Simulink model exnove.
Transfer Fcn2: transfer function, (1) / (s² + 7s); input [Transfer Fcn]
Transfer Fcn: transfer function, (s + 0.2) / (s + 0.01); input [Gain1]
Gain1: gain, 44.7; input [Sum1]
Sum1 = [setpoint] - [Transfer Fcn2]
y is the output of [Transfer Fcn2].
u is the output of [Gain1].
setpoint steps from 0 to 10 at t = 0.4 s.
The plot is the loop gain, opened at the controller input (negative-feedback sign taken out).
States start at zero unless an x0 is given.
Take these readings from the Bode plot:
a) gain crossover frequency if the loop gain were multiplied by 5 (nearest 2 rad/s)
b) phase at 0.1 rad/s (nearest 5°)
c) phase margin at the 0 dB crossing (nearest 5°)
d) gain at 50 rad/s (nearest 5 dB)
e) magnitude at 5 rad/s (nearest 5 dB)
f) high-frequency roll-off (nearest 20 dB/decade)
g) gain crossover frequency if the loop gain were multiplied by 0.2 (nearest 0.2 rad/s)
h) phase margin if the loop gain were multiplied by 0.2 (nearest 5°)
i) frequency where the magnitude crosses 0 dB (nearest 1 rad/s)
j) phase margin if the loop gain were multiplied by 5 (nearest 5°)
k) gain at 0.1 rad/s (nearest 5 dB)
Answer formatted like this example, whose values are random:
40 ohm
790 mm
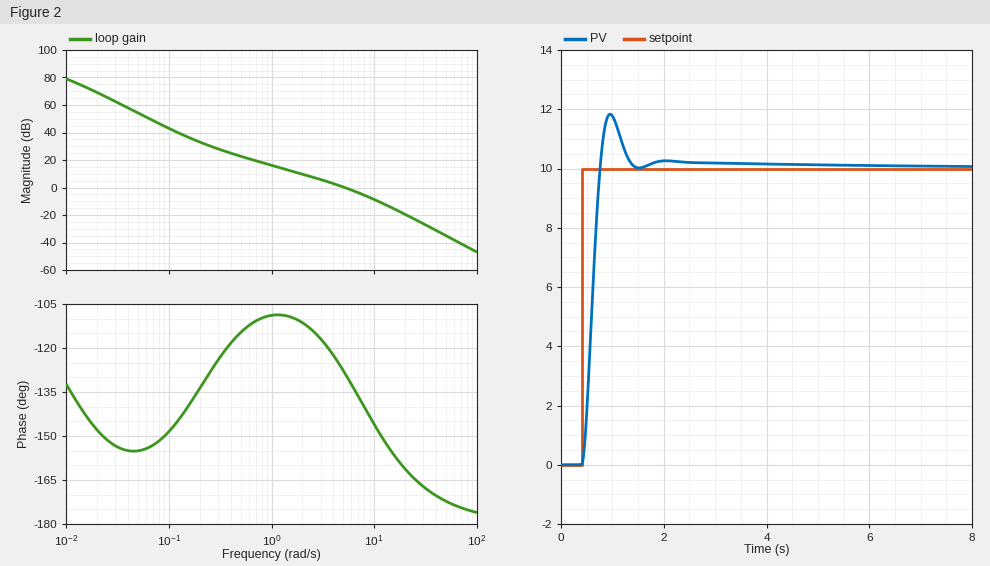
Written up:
14 rad/s
-150°
50°
-35 dB
0 dB
-40 dB/decade
1.2 rad/s
70°
5 rad/s
25°
45 dB
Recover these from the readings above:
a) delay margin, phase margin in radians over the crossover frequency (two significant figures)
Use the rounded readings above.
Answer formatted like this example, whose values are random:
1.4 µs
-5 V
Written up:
0.17 s
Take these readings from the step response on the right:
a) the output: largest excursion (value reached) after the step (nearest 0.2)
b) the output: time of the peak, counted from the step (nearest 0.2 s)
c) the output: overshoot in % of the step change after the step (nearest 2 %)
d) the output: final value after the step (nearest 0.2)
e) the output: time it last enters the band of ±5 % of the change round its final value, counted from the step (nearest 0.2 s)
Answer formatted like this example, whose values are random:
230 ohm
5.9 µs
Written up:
11.8
0.6 s
18 %
10.0
0.8 s
